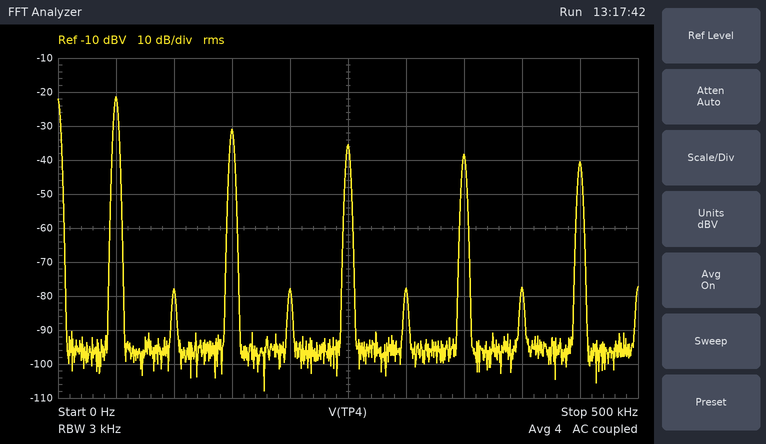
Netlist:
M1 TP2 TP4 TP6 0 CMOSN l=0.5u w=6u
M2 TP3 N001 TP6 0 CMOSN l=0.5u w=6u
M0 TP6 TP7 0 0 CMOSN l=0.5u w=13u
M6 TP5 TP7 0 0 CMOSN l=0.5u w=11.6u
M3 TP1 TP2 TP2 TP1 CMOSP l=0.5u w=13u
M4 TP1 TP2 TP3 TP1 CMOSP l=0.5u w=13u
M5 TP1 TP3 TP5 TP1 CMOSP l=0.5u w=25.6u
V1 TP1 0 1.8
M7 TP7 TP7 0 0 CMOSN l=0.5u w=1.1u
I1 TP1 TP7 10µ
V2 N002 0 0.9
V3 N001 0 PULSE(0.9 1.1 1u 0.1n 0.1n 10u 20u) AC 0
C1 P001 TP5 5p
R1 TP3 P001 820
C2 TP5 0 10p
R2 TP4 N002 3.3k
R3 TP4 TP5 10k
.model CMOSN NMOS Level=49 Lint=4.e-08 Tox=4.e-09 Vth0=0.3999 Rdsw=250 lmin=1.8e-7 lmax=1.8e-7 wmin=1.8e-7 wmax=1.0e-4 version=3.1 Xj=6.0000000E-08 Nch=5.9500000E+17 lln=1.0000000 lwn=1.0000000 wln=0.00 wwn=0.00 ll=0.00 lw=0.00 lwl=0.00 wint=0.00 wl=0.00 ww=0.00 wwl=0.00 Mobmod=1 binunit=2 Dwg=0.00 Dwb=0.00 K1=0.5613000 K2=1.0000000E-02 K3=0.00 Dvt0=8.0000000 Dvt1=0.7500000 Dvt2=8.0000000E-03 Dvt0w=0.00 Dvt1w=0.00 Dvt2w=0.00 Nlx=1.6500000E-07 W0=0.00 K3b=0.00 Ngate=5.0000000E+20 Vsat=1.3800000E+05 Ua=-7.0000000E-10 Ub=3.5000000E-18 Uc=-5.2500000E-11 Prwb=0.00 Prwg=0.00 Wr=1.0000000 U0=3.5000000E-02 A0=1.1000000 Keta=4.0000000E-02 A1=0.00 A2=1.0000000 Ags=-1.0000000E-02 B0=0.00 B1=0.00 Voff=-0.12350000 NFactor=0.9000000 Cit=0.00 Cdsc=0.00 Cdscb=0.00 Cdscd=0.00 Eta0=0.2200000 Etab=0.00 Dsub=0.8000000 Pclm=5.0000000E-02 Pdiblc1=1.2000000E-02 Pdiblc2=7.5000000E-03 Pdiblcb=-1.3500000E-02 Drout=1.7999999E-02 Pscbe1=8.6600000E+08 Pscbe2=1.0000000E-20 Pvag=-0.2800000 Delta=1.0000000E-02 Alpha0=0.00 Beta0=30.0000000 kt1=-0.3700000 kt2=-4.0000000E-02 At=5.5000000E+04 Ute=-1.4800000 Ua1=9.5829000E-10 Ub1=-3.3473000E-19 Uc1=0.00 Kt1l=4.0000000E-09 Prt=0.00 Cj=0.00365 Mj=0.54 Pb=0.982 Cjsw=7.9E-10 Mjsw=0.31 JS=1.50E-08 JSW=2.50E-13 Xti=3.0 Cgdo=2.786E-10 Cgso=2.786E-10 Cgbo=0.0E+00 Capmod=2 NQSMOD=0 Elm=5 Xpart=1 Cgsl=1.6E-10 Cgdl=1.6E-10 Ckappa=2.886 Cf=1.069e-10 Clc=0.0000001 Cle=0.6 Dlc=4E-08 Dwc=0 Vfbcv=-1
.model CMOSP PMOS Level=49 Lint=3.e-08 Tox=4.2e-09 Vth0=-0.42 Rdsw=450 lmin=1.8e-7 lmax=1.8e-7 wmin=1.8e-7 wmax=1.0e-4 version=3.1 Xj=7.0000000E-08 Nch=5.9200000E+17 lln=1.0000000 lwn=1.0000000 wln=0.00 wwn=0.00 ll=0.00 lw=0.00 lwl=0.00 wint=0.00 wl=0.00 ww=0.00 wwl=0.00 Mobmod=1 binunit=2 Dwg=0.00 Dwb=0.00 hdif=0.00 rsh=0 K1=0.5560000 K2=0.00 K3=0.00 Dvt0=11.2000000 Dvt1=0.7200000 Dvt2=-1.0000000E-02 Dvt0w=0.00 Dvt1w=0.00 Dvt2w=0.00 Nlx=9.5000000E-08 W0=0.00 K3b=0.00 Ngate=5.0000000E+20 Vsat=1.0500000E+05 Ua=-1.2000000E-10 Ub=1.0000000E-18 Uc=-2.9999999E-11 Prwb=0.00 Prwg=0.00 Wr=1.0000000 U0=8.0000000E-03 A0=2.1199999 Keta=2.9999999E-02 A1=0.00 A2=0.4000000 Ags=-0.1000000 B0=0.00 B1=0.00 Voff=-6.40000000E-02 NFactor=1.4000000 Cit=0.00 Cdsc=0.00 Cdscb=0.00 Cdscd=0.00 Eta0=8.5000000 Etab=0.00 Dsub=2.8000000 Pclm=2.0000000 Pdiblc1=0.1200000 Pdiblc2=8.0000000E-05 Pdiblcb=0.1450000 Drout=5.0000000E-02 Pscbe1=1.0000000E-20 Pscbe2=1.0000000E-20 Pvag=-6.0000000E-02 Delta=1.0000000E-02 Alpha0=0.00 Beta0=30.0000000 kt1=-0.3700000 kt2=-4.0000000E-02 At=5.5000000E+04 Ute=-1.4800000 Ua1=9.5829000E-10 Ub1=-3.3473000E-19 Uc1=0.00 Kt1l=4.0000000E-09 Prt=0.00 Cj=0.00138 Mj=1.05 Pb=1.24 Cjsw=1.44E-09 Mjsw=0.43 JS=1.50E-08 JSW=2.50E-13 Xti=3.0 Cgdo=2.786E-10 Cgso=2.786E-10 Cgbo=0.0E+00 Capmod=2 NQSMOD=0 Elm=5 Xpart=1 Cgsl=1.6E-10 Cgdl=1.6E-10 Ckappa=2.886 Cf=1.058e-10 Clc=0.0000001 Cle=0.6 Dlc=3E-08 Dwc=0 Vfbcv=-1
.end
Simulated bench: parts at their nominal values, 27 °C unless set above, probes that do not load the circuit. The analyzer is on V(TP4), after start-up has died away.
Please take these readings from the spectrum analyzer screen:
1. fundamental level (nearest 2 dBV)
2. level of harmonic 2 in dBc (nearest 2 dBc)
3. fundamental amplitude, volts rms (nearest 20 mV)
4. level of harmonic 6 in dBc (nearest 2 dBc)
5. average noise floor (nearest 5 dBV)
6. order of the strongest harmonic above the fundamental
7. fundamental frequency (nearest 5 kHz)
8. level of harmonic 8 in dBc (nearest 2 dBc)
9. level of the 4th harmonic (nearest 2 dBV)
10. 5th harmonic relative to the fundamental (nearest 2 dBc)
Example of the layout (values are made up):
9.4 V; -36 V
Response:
-22 dBV; -56 dBc; 80 mV; -56 dBc; -95 dBV; 3; 50 kHz; -56 dBc; -78 dBV; -14 dBc
